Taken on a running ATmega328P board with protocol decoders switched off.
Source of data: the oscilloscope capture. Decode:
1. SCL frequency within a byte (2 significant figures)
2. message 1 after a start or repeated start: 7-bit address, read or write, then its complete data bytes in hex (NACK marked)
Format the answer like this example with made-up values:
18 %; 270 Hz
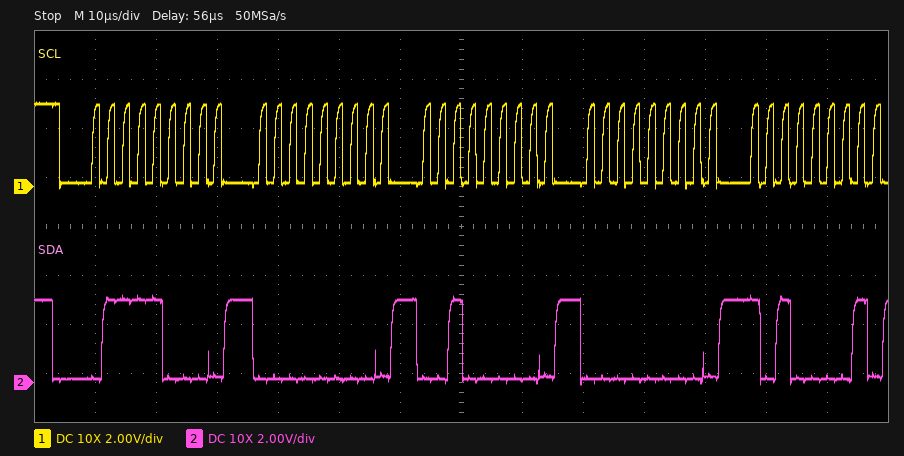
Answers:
400 kHz; 0x3C write: 00 20 00 A1
